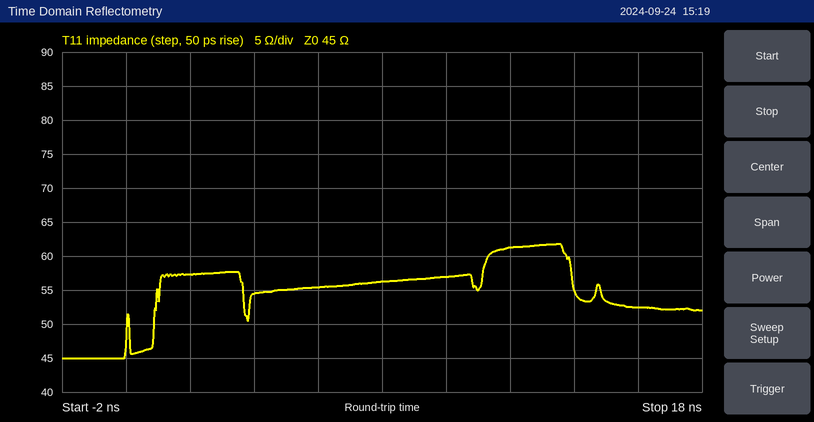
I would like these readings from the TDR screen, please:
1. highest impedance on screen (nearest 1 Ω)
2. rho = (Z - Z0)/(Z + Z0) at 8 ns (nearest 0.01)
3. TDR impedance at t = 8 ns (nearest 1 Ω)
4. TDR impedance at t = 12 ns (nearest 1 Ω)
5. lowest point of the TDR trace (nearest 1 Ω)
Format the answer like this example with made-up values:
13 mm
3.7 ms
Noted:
62 Ω
+0.11
56 Ω
61 Ω
45 Ω
